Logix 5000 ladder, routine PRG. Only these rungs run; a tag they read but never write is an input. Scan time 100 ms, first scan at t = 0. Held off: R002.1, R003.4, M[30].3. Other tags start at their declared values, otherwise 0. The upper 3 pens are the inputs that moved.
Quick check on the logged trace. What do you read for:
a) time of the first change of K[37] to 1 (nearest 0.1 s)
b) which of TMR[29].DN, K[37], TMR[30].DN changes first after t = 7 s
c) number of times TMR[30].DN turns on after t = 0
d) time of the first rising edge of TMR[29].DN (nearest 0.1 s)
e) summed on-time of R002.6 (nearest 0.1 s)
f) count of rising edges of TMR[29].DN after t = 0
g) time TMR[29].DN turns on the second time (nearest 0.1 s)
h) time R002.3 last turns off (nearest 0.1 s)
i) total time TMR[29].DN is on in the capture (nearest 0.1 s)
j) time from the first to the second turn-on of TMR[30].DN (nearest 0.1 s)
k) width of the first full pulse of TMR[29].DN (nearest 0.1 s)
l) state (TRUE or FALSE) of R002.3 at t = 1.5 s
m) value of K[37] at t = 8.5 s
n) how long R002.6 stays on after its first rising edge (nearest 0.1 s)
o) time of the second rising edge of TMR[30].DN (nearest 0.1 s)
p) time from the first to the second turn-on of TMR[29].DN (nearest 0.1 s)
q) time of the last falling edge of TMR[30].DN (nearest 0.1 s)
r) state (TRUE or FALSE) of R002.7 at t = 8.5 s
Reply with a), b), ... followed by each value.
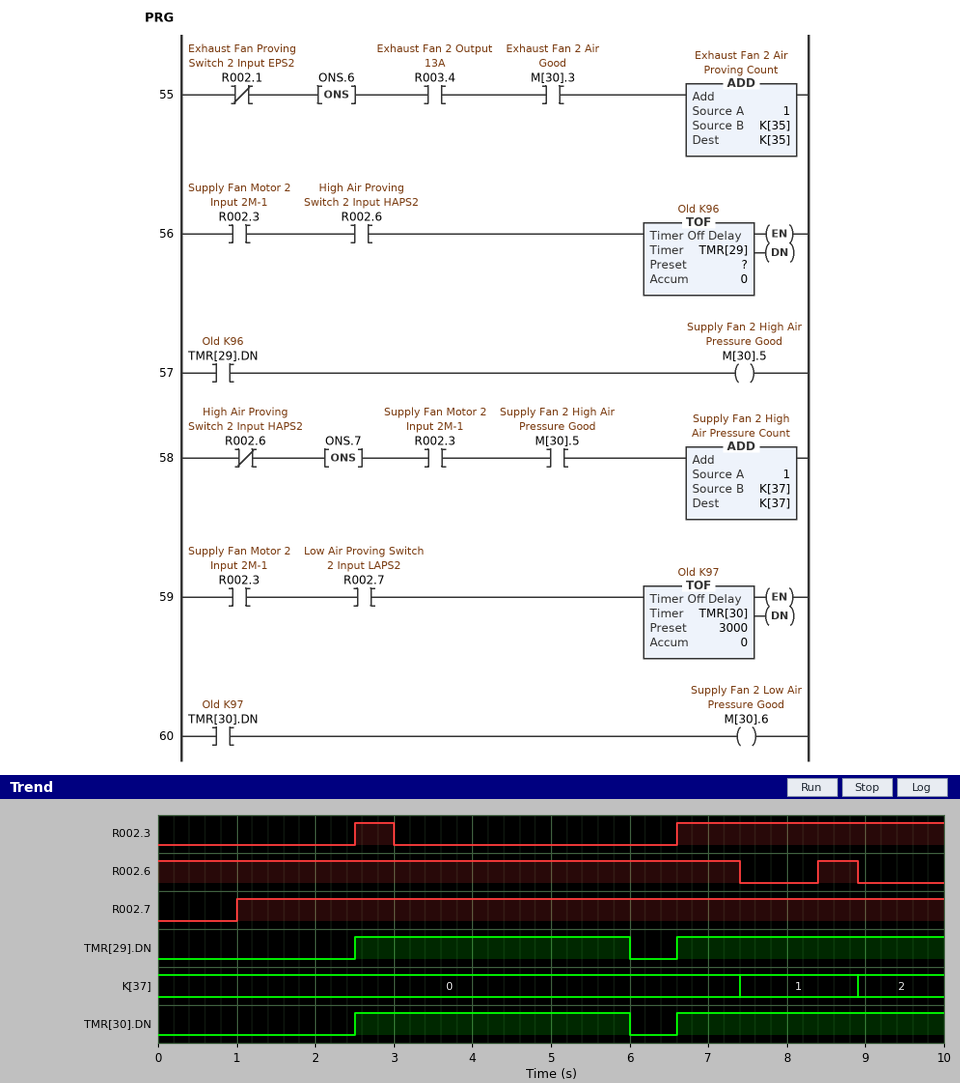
a) 7.4 s
b) K[37]
c) 2
d) 2.5 s
e) 7.9 s
f) 2
g) 6.6 s
h) 3.0 s
i) 6.9 s
j) 4.1 s
k) 3.5 s
l) FALSE
m) 1
n) 0.5 s
o) 6.6 s
p) 4.1 s
q) 6.0 s
r) TRUE
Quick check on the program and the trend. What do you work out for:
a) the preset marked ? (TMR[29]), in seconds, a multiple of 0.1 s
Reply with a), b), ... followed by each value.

a) 3.0 s
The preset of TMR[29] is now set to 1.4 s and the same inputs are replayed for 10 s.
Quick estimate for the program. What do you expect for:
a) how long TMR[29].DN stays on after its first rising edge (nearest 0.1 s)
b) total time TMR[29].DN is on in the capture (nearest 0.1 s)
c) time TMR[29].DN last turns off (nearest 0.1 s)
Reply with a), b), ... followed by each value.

a) 1.9 s
b) 5.3 s
c) 4.4 s
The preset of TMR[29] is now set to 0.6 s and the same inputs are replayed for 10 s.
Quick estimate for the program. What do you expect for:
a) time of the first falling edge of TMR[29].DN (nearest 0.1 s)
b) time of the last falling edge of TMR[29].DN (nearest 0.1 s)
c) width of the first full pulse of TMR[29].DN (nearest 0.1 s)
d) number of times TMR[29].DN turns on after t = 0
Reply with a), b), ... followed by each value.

a) 3.6 s
b) 9.5 s
c) 1.1 s
d) 3
